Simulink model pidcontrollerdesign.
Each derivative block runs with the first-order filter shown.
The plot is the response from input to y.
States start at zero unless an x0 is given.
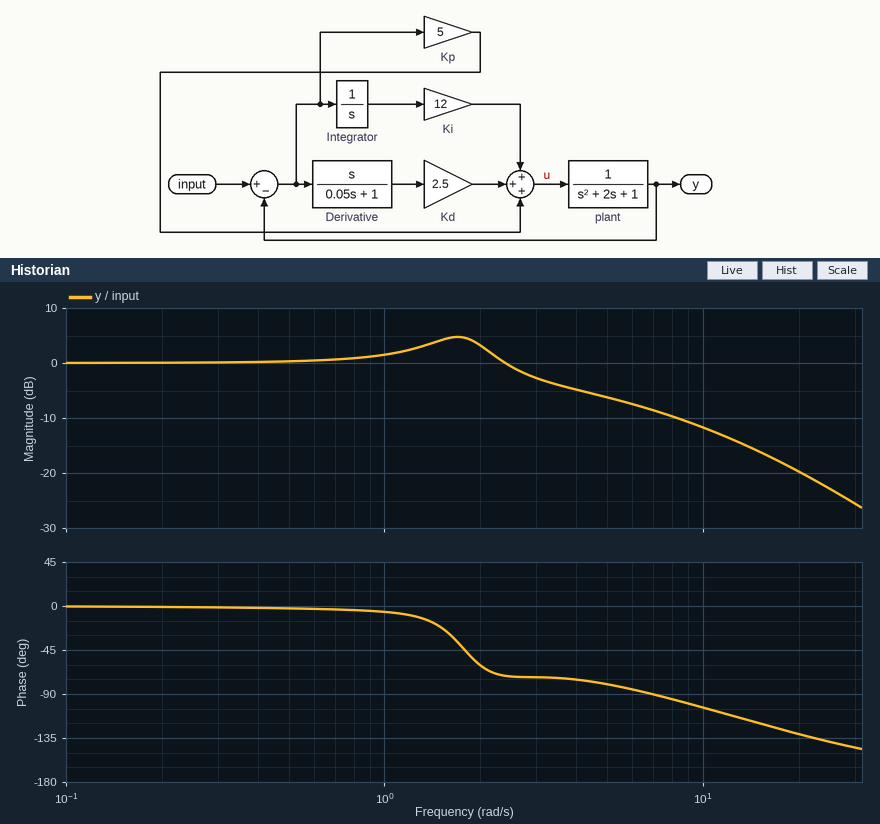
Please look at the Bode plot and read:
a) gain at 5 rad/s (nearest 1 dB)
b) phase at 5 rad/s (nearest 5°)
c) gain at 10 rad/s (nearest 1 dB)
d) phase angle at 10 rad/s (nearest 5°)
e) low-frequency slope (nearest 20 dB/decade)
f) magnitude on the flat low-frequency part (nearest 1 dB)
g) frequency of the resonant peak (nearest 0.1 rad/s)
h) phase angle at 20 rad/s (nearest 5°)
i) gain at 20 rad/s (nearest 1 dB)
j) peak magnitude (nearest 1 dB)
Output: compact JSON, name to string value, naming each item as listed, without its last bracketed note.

{"gain at 5 rad/s": "-6 dB", "phase at 5 rad/s": "-80°", "gain at 10 rad/s": "-12 dB", "phase angle at 10 rad/s": "-105°", "low-frequency slope": "0 dB/decade", "magnitude on the flat low-frequency part": "0 dB", "frequency of the resonant peak": "1.7 rad/s", "phase angle at 20 rad/s": "-130°", "gain at 20 rad/s": "-20 dB", "peak magnitude": "5 dB"}
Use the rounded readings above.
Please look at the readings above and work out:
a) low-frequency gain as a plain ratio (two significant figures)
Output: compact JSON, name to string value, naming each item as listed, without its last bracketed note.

{"low-frequency gain as a plain ratio": "1.0"}
